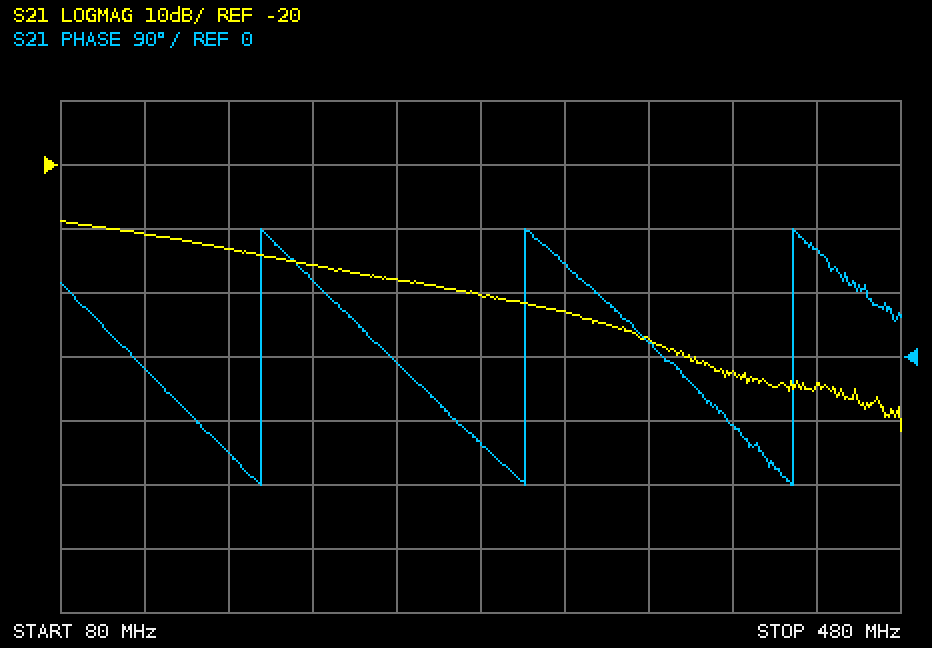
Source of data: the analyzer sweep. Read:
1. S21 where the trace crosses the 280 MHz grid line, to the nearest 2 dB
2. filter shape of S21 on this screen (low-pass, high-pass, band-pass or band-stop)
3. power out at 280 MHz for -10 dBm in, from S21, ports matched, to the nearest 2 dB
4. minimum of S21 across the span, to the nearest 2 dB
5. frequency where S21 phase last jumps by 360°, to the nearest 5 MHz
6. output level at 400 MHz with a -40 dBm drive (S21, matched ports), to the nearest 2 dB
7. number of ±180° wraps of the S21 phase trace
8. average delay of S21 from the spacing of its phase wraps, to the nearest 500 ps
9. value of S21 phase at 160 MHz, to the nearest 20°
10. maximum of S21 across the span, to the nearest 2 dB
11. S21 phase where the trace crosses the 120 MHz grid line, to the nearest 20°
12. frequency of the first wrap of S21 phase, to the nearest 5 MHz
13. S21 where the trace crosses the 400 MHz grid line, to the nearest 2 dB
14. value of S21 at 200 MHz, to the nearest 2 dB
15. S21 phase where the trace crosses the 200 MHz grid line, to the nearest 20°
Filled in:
-40 dB
low-pass
-50 dBm
-62 dB
430 MHz
-92 dBm
3
8.0 ns
-140°
-28 dB
-20°
175 MHz
-52 dB
-36 dB
100°
